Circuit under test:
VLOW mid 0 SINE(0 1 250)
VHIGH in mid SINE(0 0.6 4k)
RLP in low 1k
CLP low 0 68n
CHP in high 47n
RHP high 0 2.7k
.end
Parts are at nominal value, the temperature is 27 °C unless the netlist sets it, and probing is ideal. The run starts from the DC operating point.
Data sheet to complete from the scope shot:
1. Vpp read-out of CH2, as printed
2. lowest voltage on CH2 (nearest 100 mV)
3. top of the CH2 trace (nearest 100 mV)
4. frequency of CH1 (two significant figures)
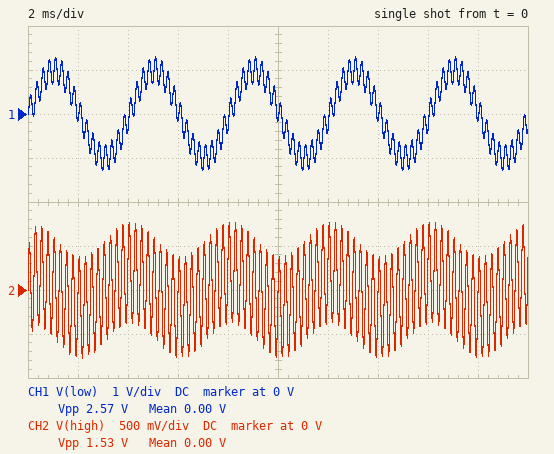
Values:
1.53 V
-800 mV
800 mV
250 Hz
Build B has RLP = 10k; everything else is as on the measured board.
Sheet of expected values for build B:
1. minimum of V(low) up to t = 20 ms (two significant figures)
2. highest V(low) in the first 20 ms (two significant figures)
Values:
-720 mV
770 mV
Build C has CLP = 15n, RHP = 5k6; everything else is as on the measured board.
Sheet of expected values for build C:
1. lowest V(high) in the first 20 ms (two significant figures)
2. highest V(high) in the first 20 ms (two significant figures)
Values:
-970 mV
970 mV
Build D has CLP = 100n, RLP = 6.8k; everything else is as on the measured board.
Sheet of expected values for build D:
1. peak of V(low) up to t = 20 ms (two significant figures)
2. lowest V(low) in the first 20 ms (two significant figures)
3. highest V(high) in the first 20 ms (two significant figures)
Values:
770 mV
-720 mV
770 mV
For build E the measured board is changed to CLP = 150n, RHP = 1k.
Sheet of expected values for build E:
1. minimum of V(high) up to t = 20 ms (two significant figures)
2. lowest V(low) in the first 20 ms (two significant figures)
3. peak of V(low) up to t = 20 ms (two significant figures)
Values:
-530 mV
-1.1 V
1.1 V
